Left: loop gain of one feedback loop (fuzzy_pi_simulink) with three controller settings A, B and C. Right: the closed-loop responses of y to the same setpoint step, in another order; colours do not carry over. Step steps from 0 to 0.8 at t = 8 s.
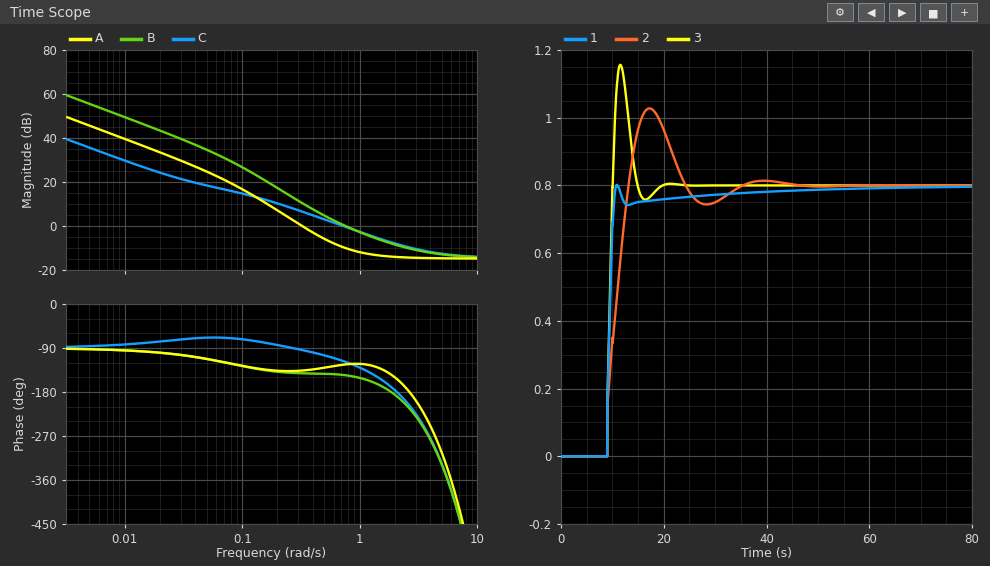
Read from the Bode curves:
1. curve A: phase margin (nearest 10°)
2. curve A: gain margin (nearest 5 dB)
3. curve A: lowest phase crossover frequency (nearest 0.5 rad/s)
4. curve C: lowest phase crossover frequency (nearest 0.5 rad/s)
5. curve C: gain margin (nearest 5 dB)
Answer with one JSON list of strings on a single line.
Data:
["40°", "15 dB", "2.5 rad/s", "2.0 rad/s", "10 dB"]
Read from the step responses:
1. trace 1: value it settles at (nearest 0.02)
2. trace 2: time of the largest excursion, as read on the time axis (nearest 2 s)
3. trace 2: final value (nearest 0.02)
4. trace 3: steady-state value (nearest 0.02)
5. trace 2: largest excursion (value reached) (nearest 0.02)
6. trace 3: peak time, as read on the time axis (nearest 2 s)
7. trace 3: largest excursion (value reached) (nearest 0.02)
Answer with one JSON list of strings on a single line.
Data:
["0.80", "18 s", "0.80", "0.80", "1.02", "12 s", "1.16"]
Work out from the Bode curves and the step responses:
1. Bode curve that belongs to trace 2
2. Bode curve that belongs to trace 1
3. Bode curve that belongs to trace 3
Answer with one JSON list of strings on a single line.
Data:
["A", "C", "B"]
